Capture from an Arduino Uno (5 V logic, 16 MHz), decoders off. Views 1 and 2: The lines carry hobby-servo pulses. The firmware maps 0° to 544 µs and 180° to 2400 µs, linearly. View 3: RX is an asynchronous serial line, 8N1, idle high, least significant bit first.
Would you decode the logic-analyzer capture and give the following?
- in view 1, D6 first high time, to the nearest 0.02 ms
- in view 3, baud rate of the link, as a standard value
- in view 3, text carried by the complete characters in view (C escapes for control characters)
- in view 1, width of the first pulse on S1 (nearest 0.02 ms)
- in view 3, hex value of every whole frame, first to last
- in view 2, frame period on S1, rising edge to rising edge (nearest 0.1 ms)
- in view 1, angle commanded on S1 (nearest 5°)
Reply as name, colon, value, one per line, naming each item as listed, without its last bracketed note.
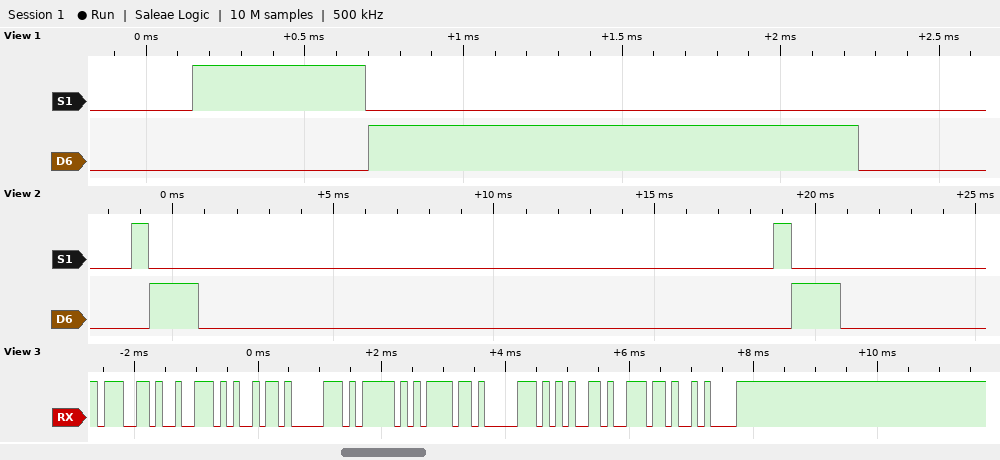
in view 1, D6 first high time, to the nearest 0.02 ms: 1.54 ms
in view 3, baud rate of the link, as a standard value: 9600 baud
in view 3, text carried by the complete characters in view: "grip_open\n"
in view 1, width of the first pulse on S1: 0.54 ms
in view 3, hex value of every whole frame, first to last: 67 72 69 70 5F 6F 70 65 6E 0A
in view 2, frame period on S1, rising edge to rising edge: 20.0 ms
in view 1, angle commanded on S1: 0°
